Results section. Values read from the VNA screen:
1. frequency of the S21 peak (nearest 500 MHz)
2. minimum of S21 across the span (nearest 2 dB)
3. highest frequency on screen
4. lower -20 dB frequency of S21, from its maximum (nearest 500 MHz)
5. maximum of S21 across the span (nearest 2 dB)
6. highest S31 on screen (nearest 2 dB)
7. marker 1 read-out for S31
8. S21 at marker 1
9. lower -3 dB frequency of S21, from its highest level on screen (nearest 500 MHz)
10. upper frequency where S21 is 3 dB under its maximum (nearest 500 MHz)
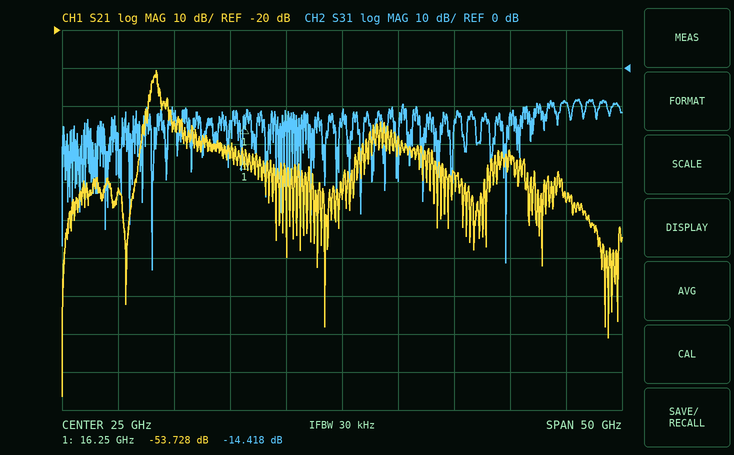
8.5 GHz
-116 dB
50 GHz
7.0 GHz
-30 dB
-8 dB
-14.418 dB
-53.728 dB
8.0 GHz
8.5 GHz
